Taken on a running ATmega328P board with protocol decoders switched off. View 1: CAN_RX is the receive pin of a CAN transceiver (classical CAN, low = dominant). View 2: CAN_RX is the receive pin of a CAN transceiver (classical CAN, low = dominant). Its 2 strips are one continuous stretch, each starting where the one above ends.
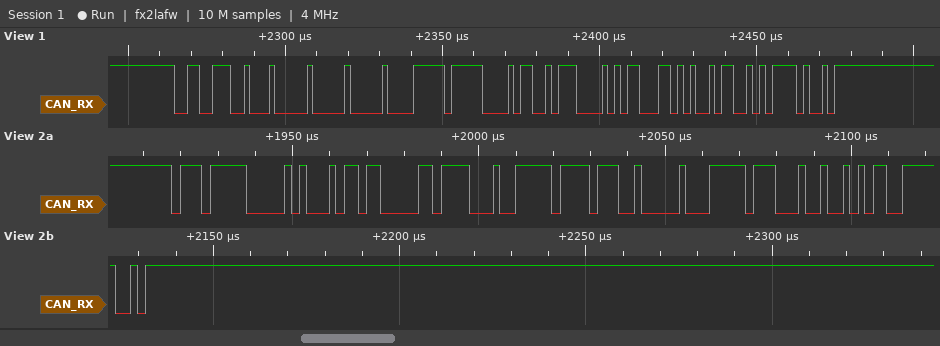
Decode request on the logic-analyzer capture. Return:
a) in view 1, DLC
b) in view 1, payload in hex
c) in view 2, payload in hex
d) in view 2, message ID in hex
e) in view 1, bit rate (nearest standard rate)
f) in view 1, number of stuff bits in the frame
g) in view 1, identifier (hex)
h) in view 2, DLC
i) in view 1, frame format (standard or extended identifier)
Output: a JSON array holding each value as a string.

["8", "00 00 FF C5 97 0A C6 A5", "B6 0B C4 FF B9 00 FF 12", "0x77C", "500 kbit/s", "5", "0x339", "8", "standard"]
